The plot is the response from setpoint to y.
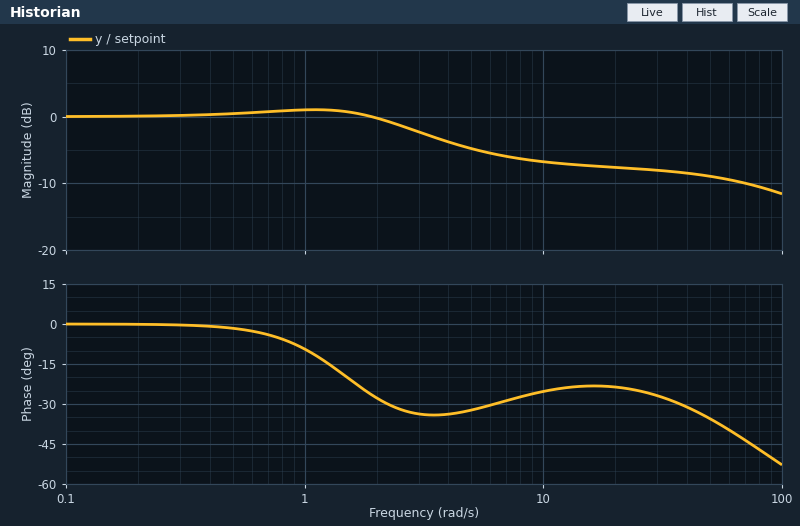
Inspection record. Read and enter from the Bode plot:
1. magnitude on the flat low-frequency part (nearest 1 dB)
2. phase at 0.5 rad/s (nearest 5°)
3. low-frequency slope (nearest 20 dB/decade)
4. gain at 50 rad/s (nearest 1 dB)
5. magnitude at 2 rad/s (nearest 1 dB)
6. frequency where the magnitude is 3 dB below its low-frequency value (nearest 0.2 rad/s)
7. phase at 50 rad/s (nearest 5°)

0 dB
0°
0 dB/decade
-9 dB
0 dB
3.4 rad/s
-35°
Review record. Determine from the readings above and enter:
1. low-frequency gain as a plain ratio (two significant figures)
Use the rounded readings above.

1.0
